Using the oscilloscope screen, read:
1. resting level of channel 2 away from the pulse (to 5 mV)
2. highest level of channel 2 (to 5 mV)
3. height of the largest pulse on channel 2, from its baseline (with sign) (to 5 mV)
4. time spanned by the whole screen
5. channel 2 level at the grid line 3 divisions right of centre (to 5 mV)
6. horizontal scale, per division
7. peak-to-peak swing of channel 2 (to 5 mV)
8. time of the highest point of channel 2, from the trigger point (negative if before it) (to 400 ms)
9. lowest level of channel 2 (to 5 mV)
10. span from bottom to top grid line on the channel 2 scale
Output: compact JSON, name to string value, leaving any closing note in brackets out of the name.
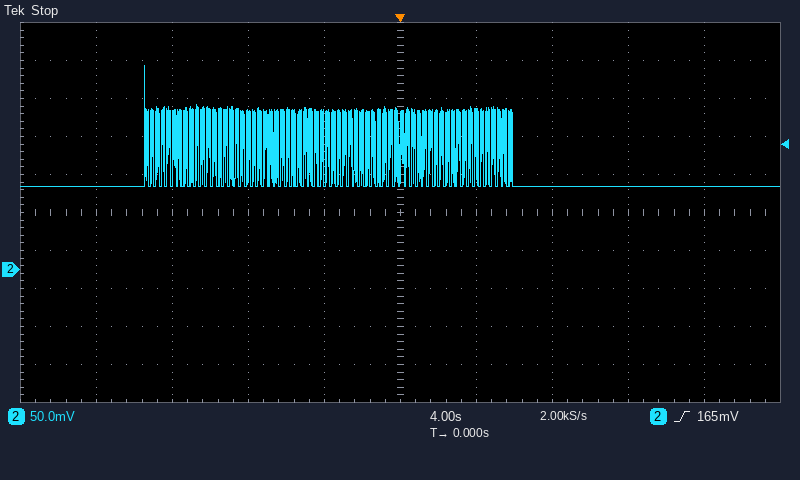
{"resting level of channel 2 away from the pulse": "110 mV", "highest level of channel 2": "270 mV", "height of the largest pulse on channel 2, from its baseline (with sign)": "+160 mV", "time spanned by the whole screen": "40 s", "channel 2 level at the grid line 3 divisions right of centre": "110 mV", "horizontal scale, per division": "4 s", "peak-to-peak swing of channel 2": "160 mV", "time of the highest point of channel 2, from the trigger point (negative if before it)": "-13.6 s", "lowest level of channel 2": "110 mV", "span from bottom to top grid line on the channel 2 scale": "500 mV"}
